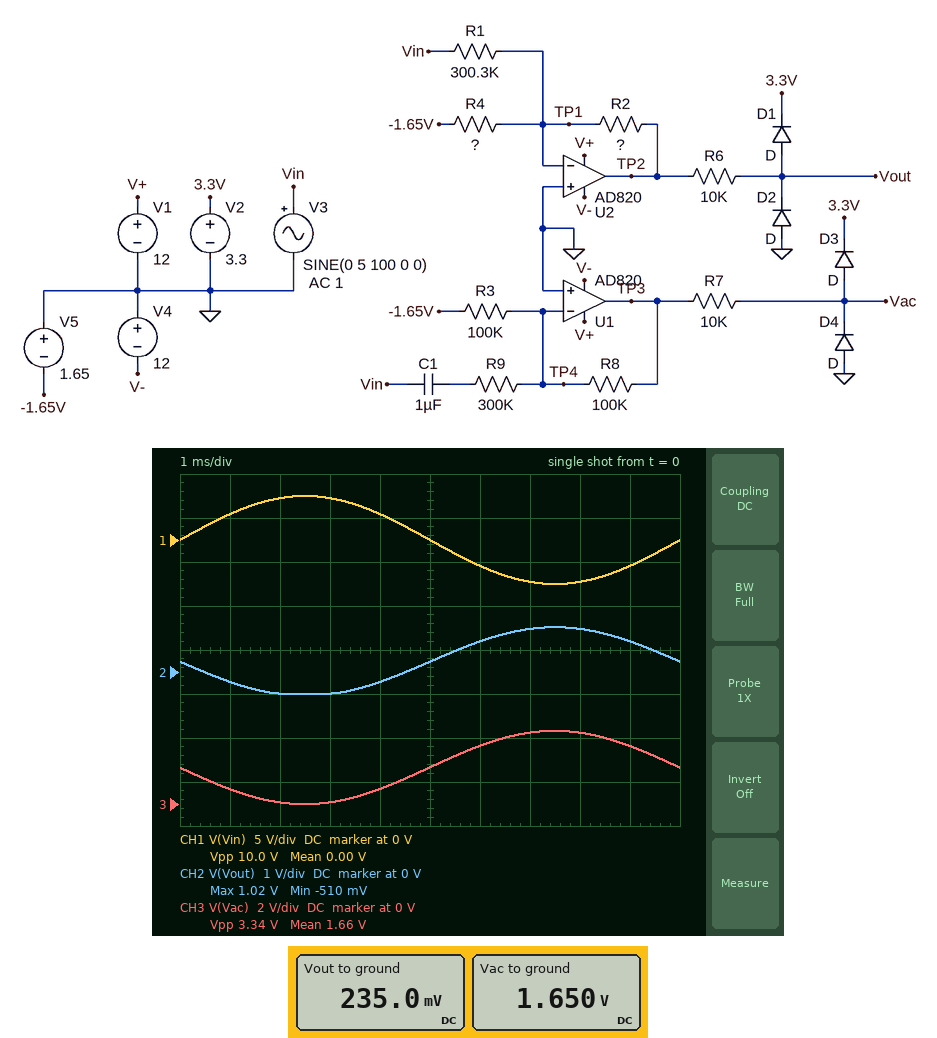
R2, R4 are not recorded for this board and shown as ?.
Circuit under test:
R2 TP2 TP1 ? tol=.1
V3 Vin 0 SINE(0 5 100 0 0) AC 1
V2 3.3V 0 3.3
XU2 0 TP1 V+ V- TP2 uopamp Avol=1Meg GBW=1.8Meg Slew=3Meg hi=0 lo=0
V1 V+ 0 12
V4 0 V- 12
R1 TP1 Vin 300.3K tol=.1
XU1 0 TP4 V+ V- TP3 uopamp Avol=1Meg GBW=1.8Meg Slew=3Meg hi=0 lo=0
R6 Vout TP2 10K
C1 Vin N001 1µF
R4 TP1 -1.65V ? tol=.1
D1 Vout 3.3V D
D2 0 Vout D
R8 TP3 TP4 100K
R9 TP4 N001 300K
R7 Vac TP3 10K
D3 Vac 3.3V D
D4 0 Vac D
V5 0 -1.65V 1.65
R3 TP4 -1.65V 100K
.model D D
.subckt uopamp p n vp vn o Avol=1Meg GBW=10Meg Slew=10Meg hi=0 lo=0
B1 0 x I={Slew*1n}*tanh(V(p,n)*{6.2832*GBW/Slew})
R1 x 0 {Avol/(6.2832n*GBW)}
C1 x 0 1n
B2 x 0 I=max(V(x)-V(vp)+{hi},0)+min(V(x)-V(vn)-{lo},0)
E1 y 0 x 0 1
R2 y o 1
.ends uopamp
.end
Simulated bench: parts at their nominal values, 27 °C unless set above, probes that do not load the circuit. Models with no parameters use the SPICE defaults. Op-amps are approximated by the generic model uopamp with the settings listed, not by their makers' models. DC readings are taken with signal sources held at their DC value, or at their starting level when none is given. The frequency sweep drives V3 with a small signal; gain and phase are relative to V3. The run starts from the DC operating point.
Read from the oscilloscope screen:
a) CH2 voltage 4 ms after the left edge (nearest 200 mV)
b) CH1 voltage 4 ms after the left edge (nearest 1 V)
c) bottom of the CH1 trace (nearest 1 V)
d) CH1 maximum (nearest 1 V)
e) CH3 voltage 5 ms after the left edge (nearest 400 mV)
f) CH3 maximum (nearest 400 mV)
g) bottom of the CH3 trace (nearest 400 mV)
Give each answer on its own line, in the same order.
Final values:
-200 mV
3 V
-5 V
5 V
1.6 V
3.2 V
0 V
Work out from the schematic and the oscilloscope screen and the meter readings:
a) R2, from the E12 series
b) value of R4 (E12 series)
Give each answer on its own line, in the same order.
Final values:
47 kΩ
330 kΩ
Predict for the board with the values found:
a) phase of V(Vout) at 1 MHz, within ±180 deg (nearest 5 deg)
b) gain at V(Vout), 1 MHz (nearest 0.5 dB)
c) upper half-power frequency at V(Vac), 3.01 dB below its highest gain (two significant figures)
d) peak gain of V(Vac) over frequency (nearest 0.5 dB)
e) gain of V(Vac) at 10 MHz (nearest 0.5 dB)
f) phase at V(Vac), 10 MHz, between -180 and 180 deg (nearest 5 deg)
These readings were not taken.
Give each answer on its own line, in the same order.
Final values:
145 deg
-18.0 dB
770 kHz
-9.5 dB
-32.0 dB
95 deg
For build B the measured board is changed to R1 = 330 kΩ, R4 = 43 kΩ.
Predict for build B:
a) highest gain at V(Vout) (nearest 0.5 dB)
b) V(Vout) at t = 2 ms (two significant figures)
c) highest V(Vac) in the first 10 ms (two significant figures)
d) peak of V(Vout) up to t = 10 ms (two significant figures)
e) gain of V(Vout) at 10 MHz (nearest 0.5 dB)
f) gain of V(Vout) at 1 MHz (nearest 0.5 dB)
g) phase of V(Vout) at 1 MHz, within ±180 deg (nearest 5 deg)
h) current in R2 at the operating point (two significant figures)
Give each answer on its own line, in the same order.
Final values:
-17.0 dB
1.1 V
3.3 V
2.5 V
-39.0 dB
-21.0 dB
130 deg
38 µA
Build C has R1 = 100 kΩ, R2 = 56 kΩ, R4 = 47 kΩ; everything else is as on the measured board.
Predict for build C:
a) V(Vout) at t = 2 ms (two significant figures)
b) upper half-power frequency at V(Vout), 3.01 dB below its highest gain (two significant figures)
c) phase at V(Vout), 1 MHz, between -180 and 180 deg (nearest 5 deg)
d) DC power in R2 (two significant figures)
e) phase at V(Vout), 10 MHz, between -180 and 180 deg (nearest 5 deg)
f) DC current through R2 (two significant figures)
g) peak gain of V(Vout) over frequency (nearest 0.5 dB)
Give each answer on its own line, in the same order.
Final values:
-550 mV
650 kHz
125 deg
69 µW
95 deg
35 µA
-5.0 dB
